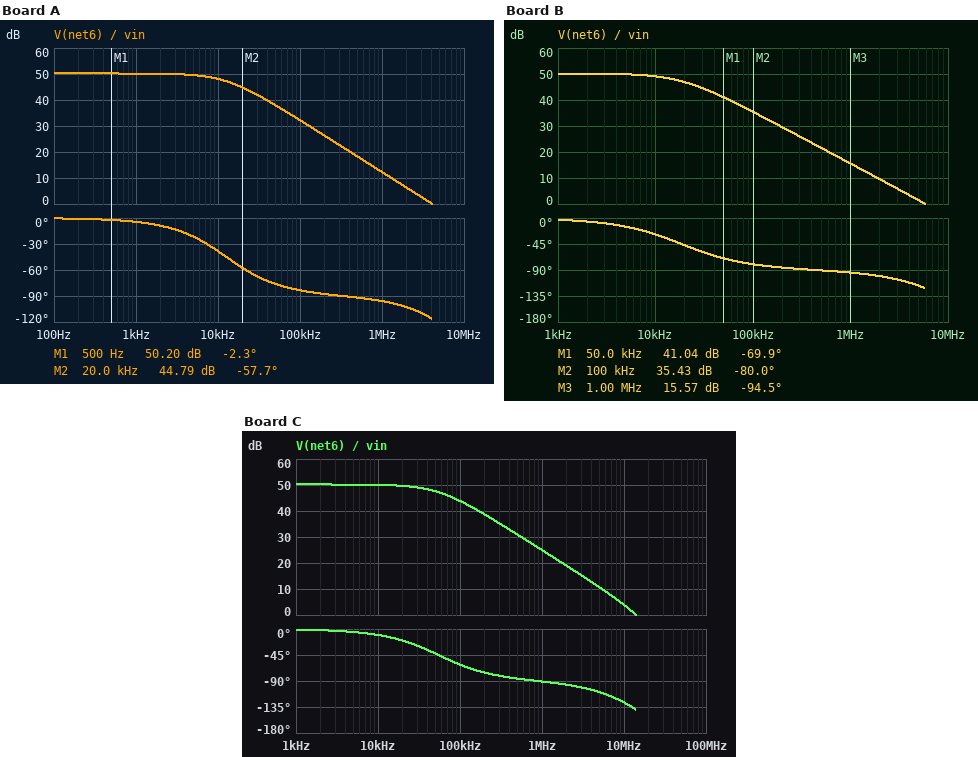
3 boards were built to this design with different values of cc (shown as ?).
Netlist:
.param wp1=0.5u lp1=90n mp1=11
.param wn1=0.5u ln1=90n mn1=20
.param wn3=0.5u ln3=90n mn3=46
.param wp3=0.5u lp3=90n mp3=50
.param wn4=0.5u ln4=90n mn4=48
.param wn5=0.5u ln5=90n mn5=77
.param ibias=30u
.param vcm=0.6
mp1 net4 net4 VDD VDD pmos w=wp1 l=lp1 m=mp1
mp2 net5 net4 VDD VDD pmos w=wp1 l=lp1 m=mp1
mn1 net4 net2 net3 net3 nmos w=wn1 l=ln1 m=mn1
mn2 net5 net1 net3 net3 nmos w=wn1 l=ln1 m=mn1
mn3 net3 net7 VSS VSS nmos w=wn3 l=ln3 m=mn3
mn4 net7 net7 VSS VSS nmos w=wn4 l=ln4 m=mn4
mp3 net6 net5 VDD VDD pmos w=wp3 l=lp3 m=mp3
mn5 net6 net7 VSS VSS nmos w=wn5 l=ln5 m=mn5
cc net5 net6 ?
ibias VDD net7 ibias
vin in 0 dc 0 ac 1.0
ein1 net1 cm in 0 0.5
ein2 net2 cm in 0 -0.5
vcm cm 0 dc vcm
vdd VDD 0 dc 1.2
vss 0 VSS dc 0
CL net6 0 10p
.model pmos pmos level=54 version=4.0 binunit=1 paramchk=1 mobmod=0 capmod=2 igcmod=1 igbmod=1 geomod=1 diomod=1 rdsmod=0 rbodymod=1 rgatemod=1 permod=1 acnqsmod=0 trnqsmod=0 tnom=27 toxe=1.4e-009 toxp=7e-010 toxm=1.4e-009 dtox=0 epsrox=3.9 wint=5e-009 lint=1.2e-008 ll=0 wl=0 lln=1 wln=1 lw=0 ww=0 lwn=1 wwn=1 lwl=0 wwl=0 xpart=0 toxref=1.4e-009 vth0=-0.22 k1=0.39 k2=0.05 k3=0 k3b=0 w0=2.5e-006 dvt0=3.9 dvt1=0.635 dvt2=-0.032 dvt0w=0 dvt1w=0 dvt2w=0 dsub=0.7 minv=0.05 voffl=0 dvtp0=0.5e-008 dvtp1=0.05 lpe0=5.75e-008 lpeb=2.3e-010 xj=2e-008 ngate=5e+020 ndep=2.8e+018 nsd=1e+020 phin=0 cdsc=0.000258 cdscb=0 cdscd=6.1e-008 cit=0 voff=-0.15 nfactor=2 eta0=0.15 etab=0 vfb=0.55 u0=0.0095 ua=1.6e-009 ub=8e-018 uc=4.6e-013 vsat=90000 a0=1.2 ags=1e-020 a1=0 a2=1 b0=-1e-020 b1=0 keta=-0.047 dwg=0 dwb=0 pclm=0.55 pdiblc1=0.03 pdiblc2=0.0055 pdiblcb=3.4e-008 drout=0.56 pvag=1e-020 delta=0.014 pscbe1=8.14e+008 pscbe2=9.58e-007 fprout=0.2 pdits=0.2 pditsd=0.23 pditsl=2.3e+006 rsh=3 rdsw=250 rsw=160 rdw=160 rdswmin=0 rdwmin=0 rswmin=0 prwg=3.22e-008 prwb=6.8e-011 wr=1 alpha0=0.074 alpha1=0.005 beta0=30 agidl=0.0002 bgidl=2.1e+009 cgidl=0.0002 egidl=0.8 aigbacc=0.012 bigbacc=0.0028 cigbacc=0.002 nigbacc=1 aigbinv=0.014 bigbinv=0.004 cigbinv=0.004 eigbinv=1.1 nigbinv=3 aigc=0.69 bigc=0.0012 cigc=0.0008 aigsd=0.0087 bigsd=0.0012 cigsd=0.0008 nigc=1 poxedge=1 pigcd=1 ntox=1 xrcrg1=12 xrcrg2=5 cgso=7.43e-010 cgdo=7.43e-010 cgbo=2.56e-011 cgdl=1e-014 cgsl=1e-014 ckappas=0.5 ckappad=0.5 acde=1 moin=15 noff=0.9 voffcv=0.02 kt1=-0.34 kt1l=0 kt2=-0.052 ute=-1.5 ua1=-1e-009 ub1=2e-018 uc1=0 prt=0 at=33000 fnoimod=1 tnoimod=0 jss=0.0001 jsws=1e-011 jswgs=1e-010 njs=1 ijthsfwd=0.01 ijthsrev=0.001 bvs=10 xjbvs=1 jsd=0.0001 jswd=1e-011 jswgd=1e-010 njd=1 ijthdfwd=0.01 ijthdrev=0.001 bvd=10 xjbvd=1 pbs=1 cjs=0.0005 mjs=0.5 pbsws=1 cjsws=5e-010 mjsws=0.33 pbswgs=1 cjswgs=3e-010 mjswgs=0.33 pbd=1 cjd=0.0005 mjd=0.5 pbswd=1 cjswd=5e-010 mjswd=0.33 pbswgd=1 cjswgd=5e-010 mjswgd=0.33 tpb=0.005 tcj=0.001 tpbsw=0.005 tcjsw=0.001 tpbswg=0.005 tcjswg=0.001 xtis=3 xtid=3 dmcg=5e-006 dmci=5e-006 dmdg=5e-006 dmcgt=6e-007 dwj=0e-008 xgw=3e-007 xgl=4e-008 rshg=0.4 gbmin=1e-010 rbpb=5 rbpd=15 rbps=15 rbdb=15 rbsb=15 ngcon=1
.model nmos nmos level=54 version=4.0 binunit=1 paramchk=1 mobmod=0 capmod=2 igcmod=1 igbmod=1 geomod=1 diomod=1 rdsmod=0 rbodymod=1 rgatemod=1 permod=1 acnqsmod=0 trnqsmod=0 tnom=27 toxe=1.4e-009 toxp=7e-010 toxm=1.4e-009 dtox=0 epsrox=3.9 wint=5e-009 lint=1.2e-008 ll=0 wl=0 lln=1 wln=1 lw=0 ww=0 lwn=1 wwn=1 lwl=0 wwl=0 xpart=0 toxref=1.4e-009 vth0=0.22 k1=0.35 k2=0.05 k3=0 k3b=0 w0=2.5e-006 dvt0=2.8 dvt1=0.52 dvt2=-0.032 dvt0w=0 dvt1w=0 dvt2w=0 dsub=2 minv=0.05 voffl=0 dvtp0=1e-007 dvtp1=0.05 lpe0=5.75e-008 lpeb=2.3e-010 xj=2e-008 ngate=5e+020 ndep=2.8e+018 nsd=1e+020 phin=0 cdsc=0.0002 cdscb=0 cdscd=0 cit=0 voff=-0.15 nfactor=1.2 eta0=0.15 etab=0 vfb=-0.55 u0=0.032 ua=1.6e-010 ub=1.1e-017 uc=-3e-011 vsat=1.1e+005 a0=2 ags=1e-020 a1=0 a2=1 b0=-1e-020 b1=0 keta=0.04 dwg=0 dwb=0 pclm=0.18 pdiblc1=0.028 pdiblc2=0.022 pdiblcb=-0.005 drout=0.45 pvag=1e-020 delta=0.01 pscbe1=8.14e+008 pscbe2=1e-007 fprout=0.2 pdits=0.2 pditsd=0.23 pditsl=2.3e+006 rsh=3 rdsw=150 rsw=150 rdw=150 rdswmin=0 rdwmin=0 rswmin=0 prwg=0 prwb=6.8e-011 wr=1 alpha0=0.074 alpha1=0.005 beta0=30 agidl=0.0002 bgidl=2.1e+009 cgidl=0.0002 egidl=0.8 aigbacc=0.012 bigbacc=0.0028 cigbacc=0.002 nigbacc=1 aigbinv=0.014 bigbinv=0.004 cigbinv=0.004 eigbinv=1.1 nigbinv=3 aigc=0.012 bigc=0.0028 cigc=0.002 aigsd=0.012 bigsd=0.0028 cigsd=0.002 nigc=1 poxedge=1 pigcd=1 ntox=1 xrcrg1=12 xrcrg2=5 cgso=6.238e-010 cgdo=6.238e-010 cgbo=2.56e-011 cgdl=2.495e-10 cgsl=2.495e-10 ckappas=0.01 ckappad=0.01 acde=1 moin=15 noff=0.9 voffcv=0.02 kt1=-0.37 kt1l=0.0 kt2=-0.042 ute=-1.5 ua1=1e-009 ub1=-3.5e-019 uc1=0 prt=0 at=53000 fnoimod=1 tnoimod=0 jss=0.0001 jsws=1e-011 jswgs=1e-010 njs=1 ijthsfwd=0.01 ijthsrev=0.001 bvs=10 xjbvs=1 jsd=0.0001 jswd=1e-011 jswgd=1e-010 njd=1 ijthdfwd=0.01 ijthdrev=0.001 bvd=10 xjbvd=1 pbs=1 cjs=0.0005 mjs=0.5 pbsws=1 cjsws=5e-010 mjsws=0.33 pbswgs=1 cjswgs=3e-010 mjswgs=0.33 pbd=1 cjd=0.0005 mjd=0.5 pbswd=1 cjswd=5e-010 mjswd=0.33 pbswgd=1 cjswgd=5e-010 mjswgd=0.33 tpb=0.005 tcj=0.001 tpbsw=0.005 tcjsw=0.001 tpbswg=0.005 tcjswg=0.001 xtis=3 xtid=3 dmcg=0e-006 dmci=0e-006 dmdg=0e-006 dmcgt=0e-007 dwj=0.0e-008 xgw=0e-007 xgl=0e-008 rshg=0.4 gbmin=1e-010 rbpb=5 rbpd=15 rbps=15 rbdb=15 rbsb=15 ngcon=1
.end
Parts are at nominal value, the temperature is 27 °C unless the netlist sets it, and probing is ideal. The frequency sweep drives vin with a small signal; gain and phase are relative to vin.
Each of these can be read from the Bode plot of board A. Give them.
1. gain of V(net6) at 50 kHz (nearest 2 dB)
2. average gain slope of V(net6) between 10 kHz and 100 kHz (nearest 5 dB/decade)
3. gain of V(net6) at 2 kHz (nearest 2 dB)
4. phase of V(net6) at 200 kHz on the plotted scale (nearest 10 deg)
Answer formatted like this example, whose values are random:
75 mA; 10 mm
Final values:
38 dB; -15 dB/decade; 50 dB; -90 deg
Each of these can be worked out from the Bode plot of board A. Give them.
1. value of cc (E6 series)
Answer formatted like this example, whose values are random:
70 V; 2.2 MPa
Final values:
10 pF
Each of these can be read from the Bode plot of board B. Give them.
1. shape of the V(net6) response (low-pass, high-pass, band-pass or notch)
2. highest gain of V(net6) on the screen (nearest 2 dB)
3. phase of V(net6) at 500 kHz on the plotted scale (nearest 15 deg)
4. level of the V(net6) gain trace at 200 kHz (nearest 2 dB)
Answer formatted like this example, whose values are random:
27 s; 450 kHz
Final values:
low-pass; 50 dB; -90 deg; 30 dB
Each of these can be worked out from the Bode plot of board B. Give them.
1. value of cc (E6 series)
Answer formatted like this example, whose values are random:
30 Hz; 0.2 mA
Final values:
6.8 pF
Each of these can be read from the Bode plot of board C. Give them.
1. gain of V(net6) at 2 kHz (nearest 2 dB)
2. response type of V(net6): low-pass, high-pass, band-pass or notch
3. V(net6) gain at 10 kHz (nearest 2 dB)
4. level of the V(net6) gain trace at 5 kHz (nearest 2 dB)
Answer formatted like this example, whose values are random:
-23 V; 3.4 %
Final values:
50 dB; low-pass; 50 dB; 50 dB
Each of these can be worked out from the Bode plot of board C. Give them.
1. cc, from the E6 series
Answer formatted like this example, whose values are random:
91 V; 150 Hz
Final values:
2.2 pF
